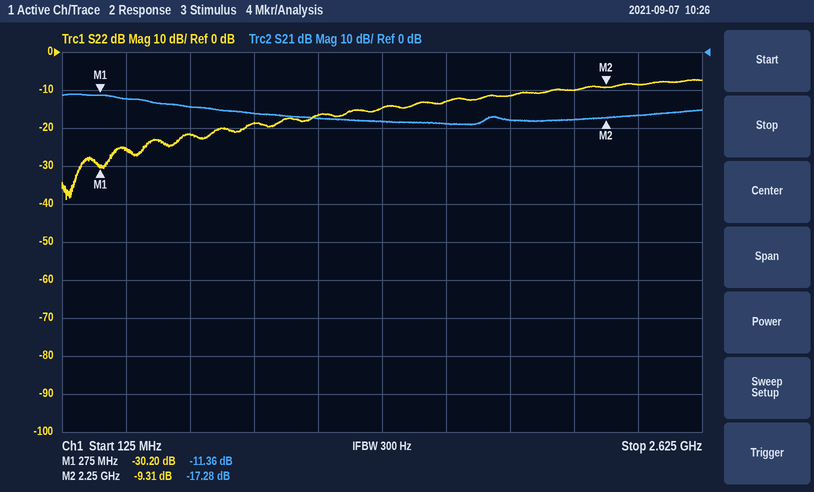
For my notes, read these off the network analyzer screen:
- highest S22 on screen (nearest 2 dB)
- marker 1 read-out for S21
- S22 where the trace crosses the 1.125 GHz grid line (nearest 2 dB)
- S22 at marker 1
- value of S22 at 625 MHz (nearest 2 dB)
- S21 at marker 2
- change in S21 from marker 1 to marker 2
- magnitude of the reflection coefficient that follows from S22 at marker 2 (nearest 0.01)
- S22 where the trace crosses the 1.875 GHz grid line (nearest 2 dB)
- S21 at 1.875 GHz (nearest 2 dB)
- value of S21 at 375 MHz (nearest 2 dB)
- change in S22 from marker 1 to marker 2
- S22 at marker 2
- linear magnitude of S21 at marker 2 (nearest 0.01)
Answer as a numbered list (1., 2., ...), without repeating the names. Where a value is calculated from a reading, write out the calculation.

1. -8 dB
2. -11.36 dB
3. -16 dB
4. -30.20 dB
5. -22 dB
6. -17.28 dB
7. -17.28 − (-11.36) = -5.92 dB
8. 10^(-9.31/20) ≈ 0.34
9. -12 dB
10. -18 dB
11. -12 dB
12. -9.31 − (-30.2) = 20.89 dB
13. -9.31 dB
14. 10^(-17.28/20) ≈ 0.14
